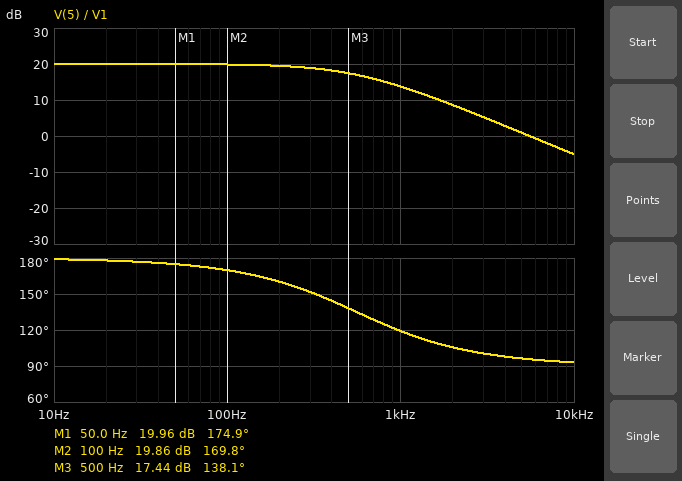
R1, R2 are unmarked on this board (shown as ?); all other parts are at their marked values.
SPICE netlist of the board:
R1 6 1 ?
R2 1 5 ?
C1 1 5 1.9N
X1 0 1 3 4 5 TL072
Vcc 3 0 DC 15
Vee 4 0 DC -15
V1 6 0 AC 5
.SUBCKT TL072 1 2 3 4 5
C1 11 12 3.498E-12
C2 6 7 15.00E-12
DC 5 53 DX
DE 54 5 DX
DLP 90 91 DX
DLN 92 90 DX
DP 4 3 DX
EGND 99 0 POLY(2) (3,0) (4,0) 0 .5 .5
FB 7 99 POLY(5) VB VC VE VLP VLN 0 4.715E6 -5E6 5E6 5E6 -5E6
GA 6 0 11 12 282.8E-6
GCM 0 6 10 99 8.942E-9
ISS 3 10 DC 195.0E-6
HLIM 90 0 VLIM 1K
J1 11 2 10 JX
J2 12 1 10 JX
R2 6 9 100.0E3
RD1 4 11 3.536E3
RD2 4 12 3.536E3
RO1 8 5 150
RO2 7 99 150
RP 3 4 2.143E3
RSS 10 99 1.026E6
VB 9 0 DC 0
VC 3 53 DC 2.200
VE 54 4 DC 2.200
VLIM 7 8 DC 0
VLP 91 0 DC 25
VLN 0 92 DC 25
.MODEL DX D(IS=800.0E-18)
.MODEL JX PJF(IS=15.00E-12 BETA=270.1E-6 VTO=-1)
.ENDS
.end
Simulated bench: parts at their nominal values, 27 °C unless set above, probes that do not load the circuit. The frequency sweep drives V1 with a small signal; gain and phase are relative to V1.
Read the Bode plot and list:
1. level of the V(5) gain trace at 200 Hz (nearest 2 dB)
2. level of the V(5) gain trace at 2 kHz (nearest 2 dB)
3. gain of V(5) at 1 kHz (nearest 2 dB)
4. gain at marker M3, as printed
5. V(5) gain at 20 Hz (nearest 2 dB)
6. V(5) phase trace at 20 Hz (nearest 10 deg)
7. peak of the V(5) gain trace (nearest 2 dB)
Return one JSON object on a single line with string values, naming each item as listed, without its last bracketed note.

{"level of the V(5) gain trace at 200 Hz": "20 dB", "level of the V(5) gain trace at 2 kHz": "8 dB", "gain of V(5) at 1 kHz": "14 dB", "gain at marker M3, as printed": "17.44 dB", "V(5) gain at 20 Hz": "20 dB", "V(5) phase trace at 20 Hz": "180 deg", "peak of the V(5) gain trace": "20 dB"}
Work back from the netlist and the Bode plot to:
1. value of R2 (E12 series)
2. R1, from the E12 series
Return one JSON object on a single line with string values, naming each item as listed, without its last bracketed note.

{"value of R2": "150 kΩ", "R1, from the E12 series": "15 kΩ"}
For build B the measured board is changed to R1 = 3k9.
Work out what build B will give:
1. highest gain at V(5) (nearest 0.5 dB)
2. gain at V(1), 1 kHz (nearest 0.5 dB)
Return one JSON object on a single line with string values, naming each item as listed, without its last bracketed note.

{"highest gain at V(5)": "31.5 dB", "gain at V(1), 1 kHz": "-45.5 dB"}
